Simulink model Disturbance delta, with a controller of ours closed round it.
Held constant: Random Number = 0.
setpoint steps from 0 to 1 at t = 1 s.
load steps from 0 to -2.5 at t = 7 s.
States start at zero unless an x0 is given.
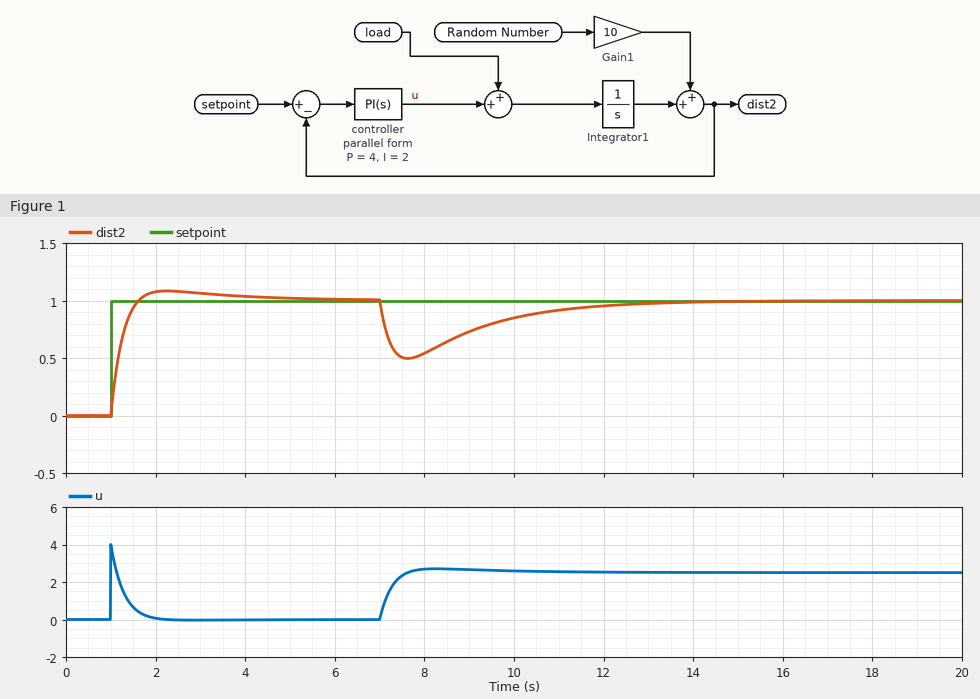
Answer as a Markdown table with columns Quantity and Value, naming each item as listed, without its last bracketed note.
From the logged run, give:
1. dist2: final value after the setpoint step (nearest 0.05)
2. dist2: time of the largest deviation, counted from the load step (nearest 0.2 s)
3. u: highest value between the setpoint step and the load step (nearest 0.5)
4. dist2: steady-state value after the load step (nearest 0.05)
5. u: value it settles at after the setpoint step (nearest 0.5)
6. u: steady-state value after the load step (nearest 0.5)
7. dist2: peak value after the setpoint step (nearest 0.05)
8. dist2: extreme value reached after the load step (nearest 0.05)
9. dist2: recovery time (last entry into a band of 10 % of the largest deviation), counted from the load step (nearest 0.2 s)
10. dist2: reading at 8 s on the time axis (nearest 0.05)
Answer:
| Quantity | Value |
|---|---|
| dist2: final value after the setpoint step | 1.00 |
| dist2: time of the largest deviation, counted from the load step | 0.6 s |
| u: highest value between the setpoint step and the load step | 4.0 |
| dist2: steady-state value after the load step | 1.00 |
| u: value it settles at after the setpoint step | 0.0 |
| u: steady-state value after the load step | 2.5 |
| dist2: peak value after the setpoint step | 1.10 |
| dist2: extreme value reached after the load step | 0.50 |
| dist2: recovery time (last entry into a band of 10 % of the largest deviation), counted from the load step | 4.8 s |
| dist2: reading at 8 s on the time axis | 0.55 |
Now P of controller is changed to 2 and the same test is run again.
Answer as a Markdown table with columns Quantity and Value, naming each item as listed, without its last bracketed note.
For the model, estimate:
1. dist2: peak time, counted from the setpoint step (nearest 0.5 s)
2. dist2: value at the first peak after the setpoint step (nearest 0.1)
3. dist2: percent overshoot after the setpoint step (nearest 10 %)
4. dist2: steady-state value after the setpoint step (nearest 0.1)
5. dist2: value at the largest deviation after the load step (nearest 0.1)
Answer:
| Quantity | Value |
|---|---|
| dist2: peak time, counted from the setpoint step | 1.5 s |
| dist2: value at the first peak after the setpoint step | 1.2 |
| dist2: percent overshoot after the setpoint step | 20 % |
| dist2: steady-state value after the setpoint step | 1.0 |
| dist2: value at the largest deviation after the load step | 0.2 |
